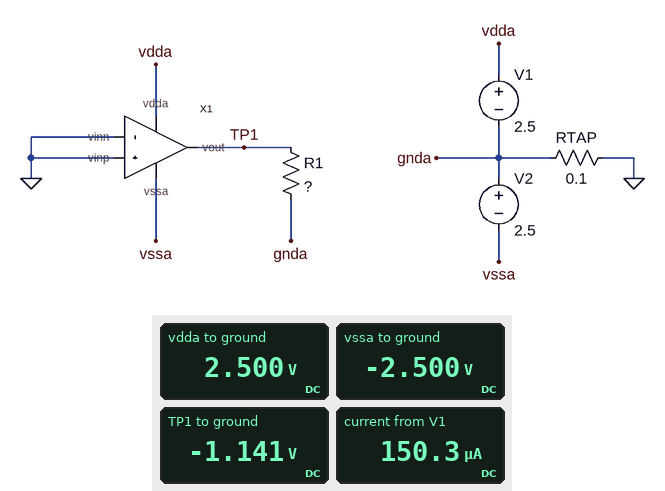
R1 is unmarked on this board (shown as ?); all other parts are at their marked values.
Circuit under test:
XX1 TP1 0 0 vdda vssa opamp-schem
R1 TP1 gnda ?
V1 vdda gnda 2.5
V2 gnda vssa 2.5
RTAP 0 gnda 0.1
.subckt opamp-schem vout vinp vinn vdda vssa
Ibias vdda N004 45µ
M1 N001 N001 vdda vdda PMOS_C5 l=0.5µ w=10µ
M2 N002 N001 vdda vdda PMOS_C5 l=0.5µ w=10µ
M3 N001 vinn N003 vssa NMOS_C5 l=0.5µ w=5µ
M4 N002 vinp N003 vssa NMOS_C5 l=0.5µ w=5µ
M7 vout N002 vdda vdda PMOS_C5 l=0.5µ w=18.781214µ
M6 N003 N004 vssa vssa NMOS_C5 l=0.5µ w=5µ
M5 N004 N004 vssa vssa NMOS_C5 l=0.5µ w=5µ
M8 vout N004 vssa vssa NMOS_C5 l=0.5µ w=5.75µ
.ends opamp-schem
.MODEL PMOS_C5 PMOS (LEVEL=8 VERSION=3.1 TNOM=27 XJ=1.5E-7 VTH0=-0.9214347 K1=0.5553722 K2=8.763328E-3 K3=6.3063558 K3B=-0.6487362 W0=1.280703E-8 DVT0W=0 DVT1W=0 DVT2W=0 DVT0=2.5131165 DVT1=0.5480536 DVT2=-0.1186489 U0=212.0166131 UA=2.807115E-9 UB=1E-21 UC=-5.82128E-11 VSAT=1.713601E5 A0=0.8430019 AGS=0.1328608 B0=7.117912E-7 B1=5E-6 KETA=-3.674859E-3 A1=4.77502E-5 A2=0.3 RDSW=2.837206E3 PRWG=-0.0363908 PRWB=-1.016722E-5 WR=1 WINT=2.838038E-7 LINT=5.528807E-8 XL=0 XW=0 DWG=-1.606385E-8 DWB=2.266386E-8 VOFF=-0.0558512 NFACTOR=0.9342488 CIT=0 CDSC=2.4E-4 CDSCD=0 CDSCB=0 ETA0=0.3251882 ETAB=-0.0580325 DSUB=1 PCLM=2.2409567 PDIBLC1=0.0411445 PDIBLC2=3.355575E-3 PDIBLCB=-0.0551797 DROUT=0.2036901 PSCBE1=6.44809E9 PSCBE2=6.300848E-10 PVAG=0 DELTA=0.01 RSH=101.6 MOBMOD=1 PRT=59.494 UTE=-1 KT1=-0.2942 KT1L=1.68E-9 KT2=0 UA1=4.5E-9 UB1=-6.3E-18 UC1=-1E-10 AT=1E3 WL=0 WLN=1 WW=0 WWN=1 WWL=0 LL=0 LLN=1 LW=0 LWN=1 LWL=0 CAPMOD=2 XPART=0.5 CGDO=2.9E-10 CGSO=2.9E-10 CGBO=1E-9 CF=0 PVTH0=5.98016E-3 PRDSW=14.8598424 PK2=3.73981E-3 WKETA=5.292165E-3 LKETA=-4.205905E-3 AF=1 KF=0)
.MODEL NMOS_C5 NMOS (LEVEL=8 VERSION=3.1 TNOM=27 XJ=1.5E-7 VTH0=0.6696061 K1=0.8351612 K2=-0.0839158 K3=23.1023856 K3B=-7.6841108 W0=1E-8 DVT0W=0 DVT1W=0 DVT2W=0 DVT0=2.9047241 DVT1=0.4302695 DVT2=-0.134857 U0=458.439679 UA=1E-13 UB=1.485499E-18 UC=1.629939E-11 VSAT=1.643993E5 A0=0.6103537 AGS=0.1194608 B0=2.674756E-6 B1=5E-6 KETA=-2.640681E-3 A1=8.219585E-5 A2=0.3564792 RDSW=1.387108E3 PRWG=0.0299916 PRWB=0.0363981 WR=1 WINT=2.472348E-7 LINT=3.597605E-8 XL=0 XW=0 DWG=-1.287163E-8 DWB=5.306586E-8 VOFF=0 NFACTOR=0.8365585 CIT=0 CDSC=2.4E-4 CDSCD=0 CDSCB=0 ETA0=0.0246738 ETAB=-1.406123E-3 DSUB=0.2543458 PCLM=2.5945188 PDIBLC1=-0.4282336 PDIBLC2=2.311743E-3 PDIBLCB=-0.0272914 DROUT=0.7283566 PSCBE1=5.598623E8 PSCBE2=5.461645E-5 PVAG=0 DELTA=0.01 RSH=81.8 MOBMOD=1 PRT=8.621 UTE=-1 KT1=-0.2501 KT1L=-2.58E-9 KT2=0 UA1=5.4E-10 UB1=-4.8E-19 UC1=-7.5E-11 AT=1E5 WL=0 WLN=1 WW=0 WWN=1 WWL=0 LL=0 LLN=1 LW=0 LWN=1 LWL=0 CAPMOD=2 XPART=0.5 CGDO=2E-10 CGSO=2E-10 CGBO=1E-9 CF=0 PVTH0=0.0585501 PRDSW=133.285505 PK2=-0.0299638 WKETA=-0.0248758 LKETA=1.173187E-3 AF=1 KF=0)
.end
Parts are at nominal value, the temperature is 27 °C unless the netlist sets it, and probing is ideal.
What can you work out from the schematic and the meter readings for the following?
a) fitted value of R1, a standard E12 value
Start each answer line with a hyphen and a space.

- 680 kΩ
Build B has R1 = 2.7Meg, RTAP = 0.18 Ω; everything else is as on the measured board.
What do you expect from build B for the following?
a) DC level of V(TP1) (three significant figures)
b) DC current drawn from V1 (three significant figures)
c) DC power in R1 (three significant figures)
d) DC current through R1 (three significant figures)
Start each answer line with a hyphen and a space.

- -1.23 V
- 151 µA
- 562 nW
- 456 nA
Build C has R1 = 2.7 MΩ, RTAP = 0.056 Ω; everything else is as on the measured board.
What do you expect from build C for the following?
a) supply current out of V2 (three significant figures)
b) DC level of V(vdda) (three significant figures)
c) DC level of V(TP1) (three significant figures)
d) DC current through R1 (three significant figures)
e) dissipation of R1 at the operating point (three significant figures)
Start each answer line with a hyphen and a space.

- 151 µA
- 2.50 V
- -1.23 V
- 456 nA
- 562 nW
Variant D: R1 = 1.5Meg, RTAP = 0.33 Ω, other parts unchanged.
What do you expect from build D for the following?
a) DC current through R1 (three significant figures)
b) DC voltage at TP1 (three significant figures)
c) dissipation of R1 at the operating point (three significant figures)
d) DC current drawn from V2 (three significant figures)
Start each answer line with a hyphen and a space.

- 804 nA
- -1.21 V
- 970 nW
- 151 µA
